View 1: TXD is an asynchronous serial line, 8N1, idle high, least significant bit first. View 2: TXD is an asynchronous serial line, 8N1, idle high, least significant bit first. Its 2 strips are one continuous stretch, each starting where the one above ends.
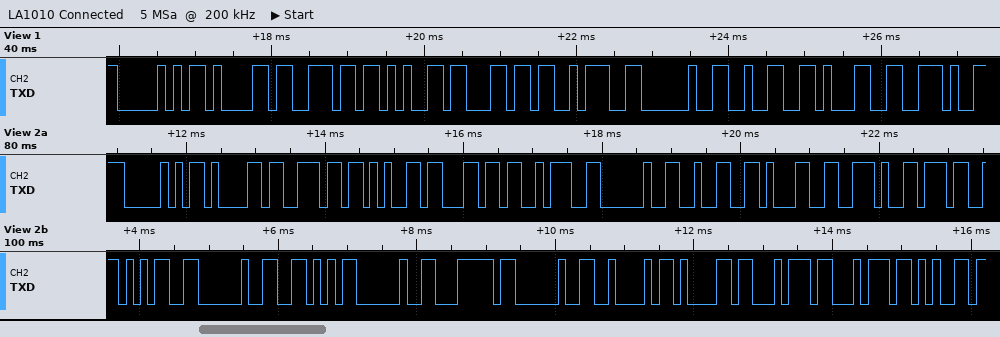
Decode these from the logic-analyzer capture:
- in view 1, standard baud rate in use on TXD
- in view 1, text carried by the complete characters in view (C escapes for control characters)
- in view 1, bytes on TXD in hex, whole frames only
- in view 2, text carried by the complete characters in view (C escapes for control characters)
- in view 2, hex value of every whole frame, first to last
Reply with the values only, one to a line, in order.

9600 baud
"Panel: 21."
0x50 0x61 0x6E 0x65 0x6C 0x3A 0x20 0x32 0x31 0x2E
"Panel: 21.75 V | Batte"
50 61 6E 65 6C 3A 20 32 31 2E 37 35 20 56 20 7C 20 42 61 74 74 65
